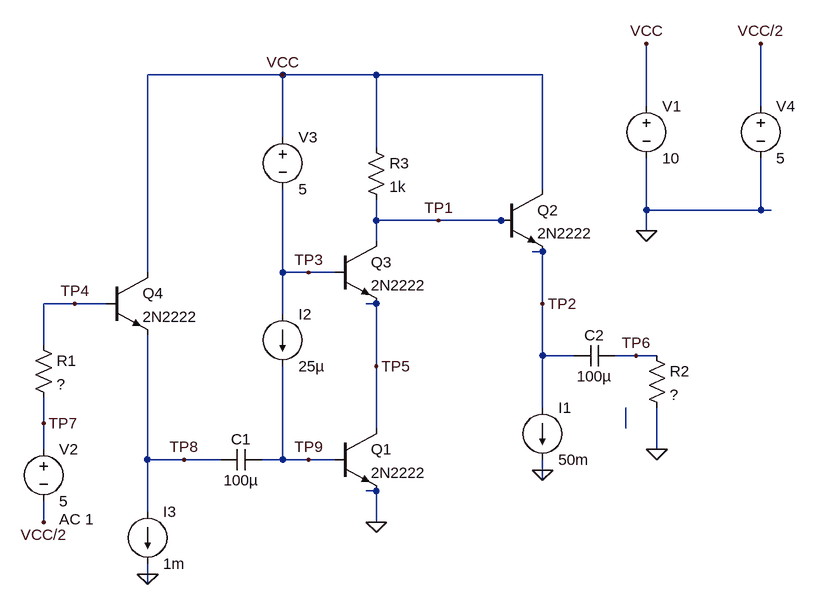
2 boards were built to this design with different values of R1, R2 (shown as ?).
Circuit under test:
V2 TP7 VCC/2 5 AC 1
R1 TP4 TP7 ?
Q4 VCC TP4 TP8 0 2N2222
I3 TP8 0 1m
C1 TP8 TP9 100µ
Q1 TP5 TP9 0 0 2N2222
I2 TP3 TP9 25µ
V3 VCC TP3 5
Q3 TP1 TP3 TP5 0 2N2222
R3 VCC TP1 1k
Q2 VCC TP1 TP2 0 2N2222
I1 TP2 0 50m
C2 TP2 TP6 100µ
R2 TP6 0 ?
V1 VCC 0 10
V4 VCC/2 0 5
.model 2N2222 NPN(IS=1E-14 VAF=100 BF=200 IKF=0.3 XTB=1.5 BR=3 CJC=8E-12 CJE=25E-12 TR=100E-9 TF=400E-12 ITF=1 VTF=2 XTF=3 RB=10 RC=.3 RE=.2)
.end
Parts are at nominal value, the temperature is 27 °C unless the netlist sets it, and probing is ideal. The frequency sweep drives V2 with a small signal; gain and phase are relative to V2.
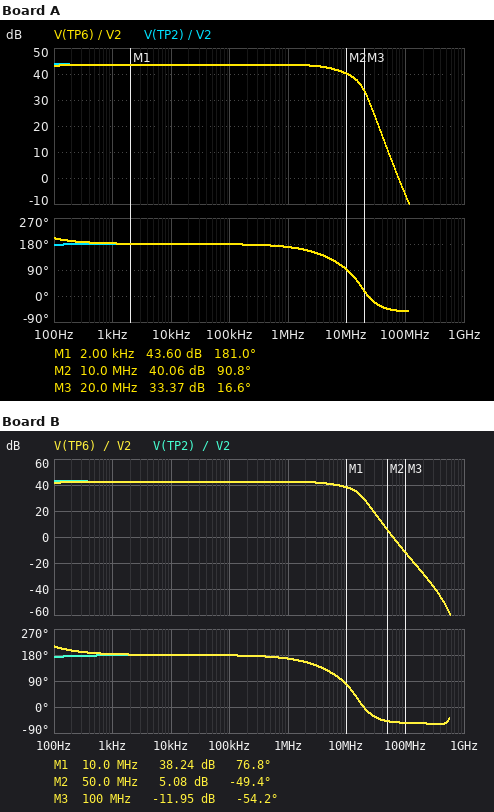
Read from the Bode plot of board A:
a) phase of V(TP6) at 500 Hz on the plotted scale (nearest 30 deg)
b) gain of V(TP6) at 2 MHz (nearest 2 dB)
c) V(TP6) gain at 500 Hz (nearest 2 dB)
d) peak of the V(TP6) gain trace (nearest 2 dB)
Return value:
180 deg
44 dB
44 dB
44 dB
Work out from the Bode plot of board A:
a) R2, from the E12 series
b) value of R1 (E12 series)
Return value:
39 Ω
330 Ω
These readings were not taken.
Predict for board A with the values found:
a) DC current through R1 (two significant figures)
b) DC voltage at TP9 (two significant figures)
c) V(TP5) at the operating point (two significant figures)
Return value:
5.0 µA
700 mV
4.3 V
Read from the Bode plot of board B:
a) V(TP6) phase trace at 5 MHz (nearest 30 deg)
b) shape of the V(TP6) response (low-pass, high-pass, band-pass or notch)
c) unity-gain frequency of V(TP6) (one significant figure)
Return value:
120 deg
low-pass
60 MHz
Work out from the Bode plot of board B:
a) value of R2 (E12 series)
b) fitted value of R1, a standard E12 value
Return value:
22 Ω
470 Ω
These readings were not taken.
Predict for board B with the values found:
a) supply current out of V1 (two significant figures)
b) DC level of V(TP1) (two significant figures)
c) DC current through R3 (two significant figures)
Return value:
56 mA
4.7 V
5.3 mA
